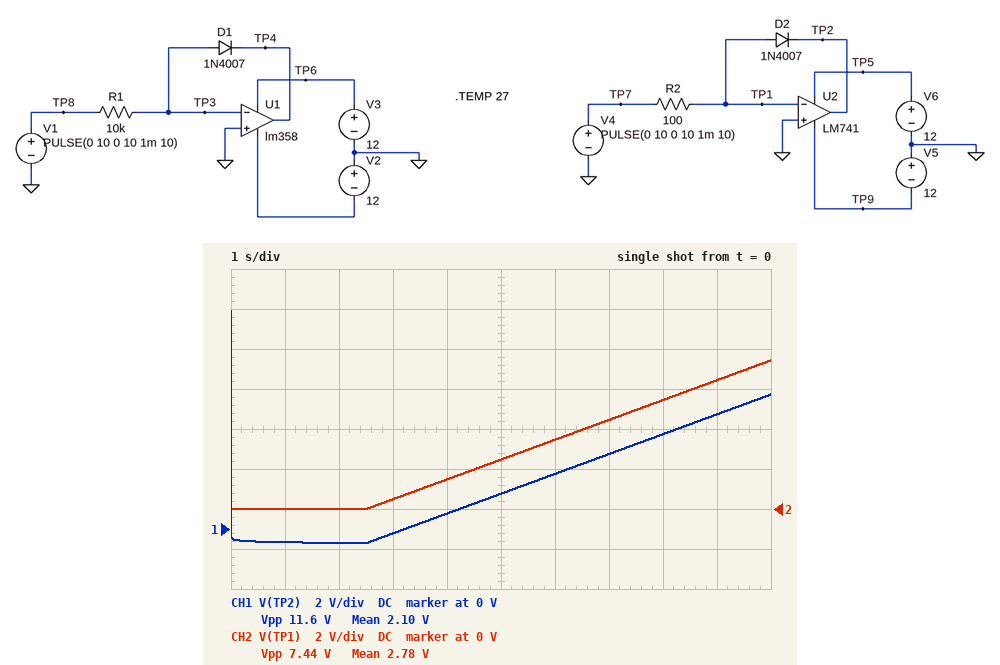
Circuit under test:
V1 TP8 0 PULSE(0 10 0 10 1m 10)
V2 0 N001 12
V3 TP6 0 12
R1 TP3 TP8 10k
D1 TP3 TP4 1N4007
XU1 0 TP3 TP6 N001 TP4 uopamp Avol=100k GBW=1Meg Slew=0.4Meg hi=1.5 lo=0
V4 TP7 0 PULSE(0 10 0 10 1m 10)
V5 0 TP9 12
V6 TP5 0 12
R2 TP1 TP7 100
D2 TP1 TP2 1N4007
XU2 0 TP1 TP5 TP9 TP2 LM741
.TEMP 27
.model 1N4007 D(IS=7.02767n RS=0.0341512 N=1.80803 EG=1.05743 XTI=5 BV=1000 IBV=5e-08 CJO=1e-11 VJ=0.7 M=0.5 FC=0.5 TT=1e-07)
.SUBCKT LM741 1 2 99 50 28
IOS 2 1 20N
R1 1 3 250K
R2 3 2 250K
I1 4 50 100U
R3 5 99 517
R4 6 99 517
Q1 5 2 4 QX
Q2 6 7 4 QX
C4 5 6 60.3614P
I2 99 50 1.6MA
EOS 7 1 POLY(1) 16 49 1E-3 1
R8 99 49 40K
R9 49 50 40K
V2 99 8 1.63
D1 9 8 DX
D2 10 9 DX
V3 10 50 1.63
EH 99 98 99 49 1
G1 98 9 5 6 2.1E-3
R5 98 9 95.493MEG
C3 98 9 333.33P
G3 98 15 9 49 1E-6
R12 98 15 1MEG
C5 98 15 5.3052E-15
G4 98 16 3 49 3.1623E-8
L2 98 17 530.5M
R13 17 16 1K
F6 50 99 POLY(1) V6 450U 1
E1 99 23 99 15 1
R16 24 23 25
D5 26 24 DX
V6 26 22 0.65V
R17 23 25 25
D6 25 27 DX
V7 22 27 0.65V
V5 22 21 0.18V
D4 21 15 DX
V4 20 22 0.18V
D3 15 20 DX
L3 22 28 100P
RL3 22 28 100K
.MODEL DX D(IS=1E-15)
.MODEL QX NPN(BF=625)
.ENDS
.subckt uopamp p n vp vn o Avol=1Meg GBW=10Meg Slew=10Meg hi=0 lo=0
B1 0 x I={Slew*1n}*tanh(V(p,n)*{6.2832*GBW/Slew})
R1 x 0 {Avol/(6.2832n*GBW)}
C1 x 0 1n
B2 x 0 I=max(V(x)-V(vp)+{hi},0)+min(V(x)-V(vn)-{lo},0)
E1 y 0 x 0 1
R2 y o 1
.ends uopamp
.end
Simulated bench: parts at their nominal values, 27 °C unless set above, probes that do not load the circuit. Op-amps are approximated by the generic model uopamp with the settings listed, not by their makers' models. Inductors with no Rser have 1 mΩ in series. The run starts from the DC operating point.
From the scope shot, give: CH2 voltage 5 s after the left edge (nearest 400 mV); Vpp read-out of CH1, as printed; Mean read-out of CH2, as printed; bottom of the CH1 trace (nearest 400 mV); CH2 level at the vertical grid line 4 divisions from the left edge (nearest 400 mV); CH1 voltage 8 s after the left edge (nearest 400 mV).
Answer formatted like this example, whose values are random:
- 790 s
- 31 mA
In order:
- 2.4 V
- 11.6 V
- 2.78 V
- -800 mV
- 1.6 V
- 4.8 V
